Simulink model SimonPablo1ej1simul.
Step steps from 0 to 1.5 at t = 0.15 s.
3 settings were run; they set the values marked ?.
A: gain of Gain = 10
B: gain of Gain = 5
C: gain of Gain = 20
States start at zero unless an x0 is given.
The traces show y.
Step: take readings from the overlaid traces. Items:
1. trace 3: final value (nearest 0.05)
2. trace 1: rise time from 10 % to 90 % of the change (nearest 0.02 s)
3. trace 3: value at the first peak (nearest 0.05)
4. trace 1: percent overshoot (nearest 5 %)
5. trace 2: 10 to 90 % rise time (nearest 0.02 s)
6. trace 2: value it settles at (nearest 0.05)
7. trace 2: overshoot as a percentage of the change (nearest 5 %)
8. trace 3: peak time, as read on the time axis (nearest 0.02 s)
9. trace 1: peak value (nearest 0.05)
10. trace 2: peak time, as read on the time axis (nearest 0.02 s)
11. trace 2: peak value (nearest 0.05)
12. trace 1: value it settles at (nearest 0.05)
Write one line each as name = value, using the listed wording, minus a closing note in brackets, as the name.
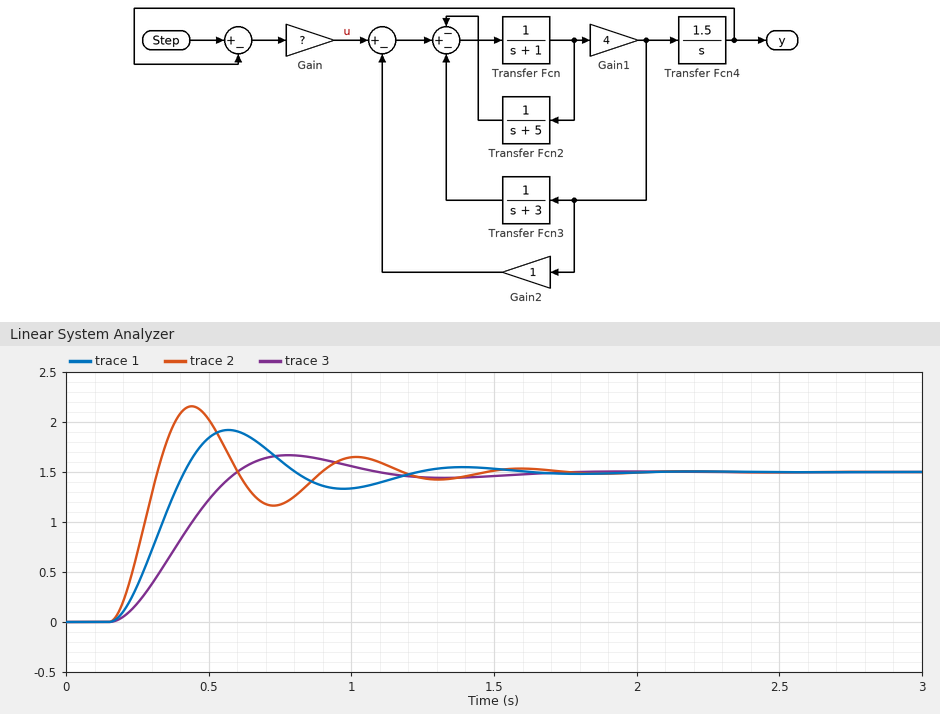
trace 3: final value = 1.50
trace 1: rise time from 10 % to 90 % of the change = 0.18 s
trace 3: value at the first peak = 1.65
trace 1: percent overshoot = 30 %
trace 2: 10 to 90 % rise time = 0.12 s
trace 2: value it settles at = 1.50
trace 2: overshoot as a percentage of the change = 45 %
trace 3: peak time, as read on the time axis = 0.78 s
trace 1: peak value = 1.90
trace 2: peak time, as read on the time axis = 0.44 s
trace 2: peak value = 2.15
trace 1: value it settles at = 1.50
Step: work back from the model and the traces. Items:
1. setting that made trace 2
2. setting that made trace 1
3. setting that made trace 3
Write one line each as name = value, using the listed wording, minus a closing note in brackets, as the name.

setting that made trace 2 = C
setting that made trace 1 = A
setting that made trace 3 = B
